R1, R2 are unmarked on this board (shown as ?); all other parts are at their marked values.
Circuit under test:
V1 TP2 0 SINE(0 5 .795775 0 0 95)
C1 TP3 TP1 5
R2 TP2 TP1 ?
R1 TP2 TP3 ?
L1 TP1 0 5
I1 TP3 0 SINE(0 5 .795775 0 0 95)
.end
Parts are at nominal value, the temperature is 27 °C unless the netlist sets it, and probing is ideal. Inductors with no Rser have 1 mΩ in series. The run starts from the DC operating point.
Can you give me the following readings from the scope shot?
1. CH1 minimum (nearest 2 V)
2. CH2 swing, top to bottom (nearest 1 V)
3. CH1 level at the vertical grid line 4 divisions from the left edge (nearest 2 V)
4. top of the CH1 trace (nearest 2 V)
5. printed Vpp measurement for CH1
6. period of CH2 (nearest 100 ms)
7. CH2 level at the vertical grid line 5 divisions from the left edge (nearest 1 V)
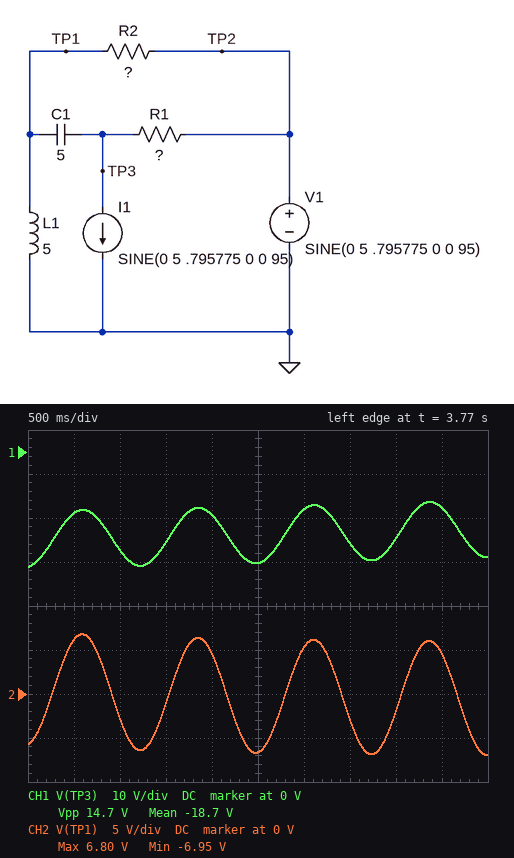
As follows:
-26 V
14 V
-14 V
-12 V
14.7 V
1.3 s
-7 V
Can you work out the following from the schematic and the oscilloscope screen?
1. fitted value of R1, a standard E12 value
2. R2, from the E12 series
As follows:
5.6 Ω
3.9 Ω
